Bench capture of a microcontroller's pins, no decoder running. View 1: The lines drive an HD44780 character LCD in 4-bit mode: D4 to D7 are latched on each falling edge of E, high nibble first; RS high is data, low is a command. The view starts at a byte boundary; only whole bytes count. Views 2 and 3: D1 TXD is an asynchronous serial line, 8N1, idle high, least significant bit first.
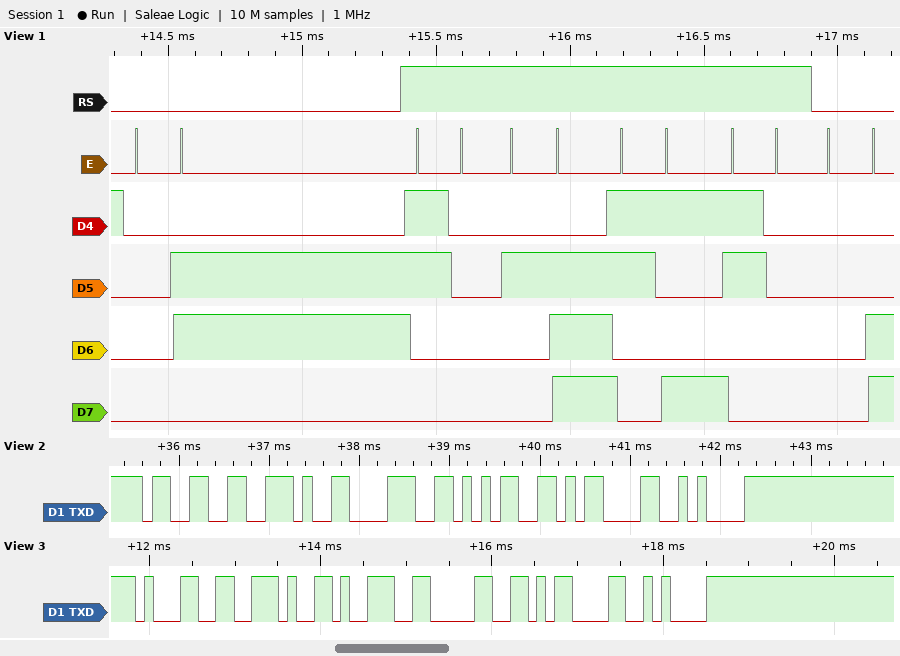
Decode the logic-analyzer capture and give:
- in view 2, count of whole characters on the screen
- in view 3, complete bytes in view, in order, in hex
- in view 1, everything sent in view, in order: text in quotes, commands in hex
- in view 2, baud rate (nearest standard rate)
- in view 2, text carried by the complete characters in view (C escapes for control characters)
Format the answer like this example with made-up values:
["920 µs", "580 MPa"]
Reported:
["6", "31 2E 39 30 0D 0A", "0x06 \"0.90\" 0x0C", "9600 baud", "\"3.85\\r\\n\""]
